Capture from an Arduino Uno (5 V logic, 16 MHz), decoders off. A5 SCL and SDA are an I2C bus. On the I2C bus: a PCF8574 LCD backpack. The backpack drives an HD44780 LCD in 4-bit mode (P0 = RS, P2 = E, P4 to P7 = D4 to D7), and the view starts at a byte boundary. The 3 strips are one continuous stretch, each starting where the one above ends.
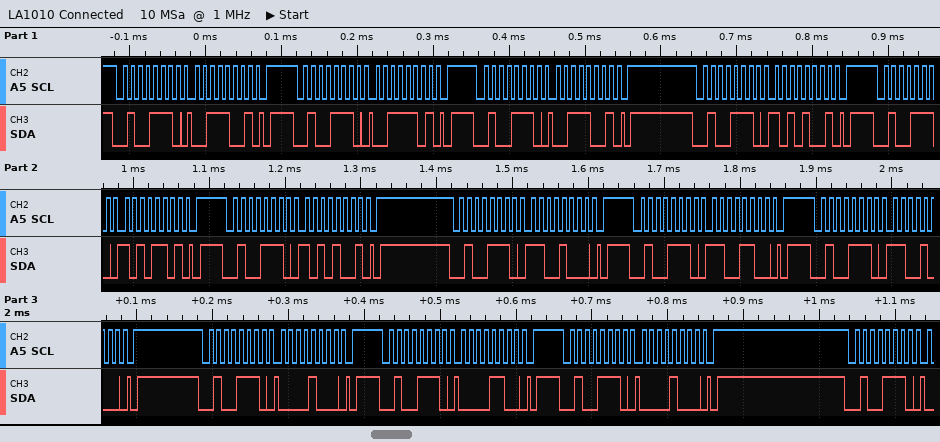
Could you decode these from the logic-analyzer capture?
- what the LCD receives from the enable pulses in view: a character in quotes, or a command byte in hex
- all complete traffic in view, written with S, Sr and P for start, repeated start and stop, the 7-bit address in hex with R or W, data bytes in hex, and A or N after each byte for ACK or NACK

':' 0xC0
S 27W A 39 A P S 27W A 3D A P S 27W A 39 A P S 27W A A9 A P S 27W A AD A P S 27W A A9 A P S 27W A C8 A P S 27W A CC A P S 27W A C8 A P S 27W A 08 A P S 27W A 0C A P S 27W A 08 A P S 27W A
